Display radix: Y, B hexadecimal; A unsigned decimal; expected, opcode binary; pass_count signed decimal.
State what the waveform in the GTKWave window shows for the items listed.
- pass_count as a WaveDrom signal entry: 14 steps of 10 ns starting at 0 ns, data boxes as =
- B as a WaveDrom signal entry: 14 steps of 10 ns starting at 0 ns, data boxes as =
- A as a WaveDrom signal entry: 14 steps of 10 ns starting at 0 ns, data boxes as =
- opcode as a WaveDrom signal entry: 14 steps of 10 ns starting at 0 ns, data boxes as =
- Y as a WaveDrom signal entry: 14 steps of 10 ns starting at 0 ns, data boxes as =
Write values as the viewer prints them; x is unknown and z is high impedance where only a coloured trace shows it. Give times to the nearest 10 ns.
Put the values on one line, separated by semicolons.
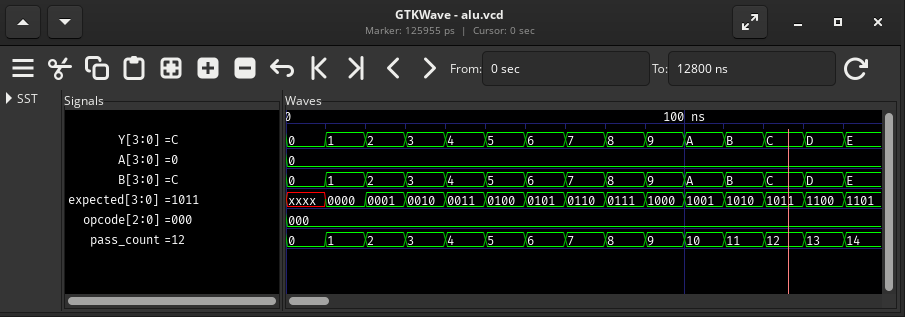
{name: 'pass_count', wave: '==============', data: '0 1 2 3 4 5 6 7 8 9 10 11 12 13'}; {name: 'B', wave: '==============', data: '0 1 2 3 4 5 6 7 8 9 A B C D'}; {name: 'A', wave: '=.............', data: '0'}; {name: 'opcode', wave: '=.............', data: '000'}; {name: 'Y', wave: '==============', data: '0 1 2 3 4 5 6 7 8 9 A B C D'}
